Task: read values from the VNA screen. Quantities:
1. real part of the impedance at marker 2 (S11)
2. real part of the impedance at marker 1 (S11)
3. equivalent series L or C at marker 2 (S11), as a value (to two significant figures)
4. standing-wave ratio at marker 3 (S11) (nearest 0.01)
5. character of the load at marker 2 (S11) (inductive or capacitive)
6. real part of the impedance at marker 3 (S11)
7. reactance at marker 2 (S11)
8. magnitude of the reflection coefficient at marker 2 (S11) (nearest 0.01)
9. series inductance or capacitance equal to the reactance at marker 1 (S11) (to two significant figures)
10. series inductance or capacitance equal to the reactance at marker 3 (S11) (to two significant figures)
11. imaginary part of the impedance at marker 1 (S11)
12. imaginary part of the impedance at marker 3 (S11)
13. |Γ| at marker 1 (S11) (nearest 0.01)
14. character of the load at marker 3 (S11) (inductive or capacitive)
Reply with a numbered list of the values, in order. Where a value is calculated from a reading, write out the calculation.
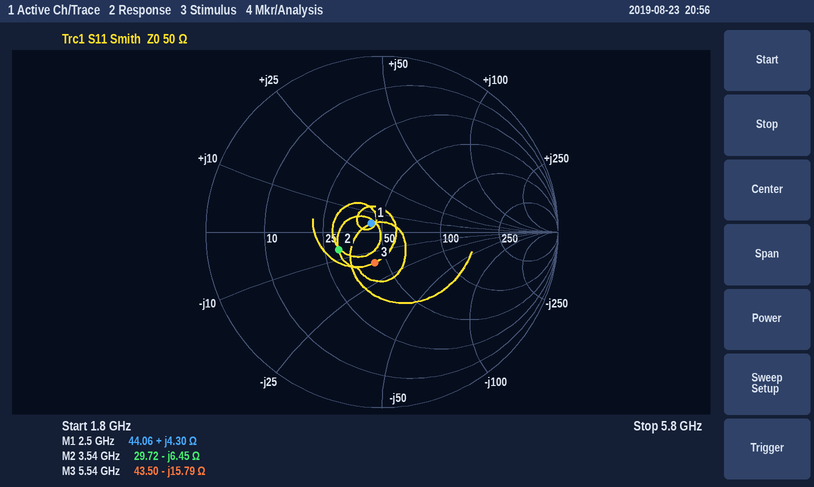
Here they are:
1. 29.72 Ω
2. 44.06 Ω
3. C = 1/(2π × 3.54 GHz × 6.45 Ω) ≈ 7.0 pF
4. 1.44
5. capacitive
6. 43.50 Ω
7. -6.45 Ω
8. 0.27
9. L = 4.3 Ω/(2π × 2.5 GHz) ≈ 274 pH, so 270 pH to two significant figures
10. C = 1/(2π × 5.54 GHz × 15.79 Ω) ≈ 1.8 pF
11. +4.30 Ω
12. -15.79 Ω
13. 0.08
14. capacitive
